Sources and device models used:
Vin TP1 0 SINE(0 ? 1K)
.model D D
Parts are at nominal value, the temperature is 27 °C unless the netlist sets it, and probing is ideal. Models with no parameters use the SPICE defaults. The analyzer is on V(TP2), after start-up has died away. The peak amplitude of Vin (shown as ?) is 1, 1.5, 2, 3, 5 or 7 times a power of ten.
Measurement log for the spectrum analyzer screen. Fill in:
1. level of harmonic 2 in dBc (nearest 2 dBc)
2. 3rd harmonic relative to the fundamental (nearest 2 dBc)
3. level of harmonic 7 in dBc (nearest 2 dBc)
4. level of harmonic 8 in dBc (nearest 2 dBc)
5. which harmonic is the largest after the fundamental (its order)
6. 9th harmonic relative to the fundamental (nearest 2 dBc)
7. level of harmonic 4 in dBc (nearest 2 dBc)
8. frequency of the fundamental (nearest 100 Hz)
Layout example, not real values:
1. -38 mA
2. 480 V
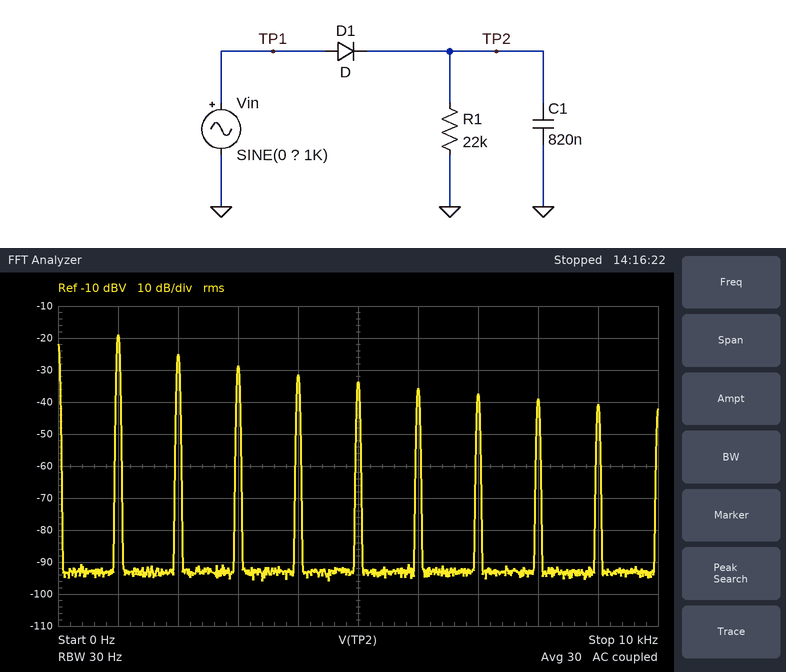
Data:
1. -6 dBc
2. -10 dBc
3. -18 dBc
4. -20 dBc
5. 2
6. -22 dBc
7. -12 dBc
8. 1.0 kHz
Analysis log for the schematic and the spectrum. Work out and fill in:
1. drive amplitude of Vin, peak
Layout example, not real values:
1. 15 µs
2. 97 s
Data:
1. 10 V
